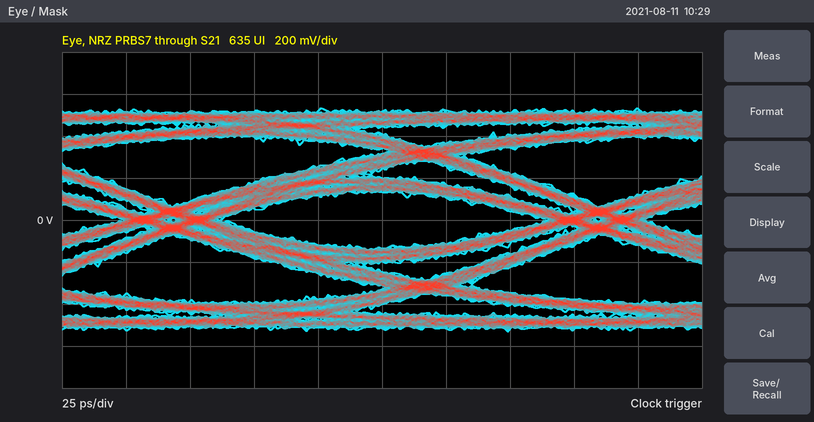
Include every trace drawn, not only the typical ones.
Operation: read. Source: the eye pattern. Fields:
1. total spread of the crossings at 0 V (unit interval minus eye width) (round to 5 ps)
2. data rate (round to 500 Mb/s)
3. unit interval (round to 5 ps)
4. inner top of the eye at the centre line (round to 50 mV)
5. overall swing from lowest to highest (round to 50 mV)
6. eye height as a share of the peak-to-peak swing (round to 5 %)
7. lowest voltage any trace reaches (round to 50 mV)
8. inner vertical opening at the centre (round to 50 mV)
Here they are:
40 ps
6.0 Gb/s
165 ps
150 mV
1.05 V
25 %
-550 mV
250 mV
